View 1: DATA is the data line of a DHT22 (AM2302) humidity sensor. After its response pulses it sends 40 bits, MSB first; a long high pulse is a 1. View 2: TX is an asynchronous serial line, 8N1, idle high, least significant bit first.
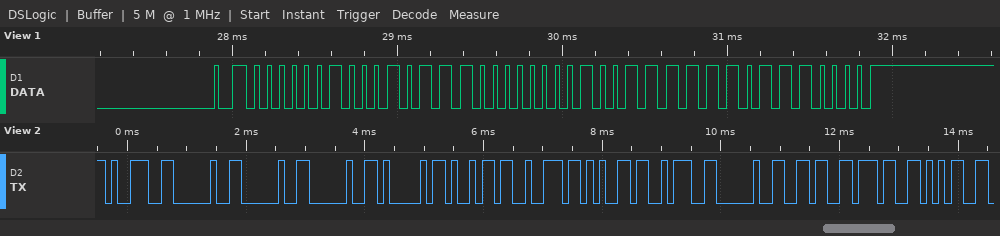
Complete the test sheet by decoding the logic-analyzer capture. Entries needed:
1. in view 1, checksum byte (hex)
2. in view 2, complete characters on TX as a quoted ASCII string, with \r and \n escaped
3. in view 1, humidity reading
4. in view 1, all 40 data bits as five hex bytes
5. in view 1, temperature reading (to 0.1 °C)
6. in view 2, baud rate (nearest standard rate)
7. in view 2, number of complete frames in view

0x70
"9   Aire: 675"
55.8 %
02 2E 01 3F 70
31.9 °C
9600 baud
13
